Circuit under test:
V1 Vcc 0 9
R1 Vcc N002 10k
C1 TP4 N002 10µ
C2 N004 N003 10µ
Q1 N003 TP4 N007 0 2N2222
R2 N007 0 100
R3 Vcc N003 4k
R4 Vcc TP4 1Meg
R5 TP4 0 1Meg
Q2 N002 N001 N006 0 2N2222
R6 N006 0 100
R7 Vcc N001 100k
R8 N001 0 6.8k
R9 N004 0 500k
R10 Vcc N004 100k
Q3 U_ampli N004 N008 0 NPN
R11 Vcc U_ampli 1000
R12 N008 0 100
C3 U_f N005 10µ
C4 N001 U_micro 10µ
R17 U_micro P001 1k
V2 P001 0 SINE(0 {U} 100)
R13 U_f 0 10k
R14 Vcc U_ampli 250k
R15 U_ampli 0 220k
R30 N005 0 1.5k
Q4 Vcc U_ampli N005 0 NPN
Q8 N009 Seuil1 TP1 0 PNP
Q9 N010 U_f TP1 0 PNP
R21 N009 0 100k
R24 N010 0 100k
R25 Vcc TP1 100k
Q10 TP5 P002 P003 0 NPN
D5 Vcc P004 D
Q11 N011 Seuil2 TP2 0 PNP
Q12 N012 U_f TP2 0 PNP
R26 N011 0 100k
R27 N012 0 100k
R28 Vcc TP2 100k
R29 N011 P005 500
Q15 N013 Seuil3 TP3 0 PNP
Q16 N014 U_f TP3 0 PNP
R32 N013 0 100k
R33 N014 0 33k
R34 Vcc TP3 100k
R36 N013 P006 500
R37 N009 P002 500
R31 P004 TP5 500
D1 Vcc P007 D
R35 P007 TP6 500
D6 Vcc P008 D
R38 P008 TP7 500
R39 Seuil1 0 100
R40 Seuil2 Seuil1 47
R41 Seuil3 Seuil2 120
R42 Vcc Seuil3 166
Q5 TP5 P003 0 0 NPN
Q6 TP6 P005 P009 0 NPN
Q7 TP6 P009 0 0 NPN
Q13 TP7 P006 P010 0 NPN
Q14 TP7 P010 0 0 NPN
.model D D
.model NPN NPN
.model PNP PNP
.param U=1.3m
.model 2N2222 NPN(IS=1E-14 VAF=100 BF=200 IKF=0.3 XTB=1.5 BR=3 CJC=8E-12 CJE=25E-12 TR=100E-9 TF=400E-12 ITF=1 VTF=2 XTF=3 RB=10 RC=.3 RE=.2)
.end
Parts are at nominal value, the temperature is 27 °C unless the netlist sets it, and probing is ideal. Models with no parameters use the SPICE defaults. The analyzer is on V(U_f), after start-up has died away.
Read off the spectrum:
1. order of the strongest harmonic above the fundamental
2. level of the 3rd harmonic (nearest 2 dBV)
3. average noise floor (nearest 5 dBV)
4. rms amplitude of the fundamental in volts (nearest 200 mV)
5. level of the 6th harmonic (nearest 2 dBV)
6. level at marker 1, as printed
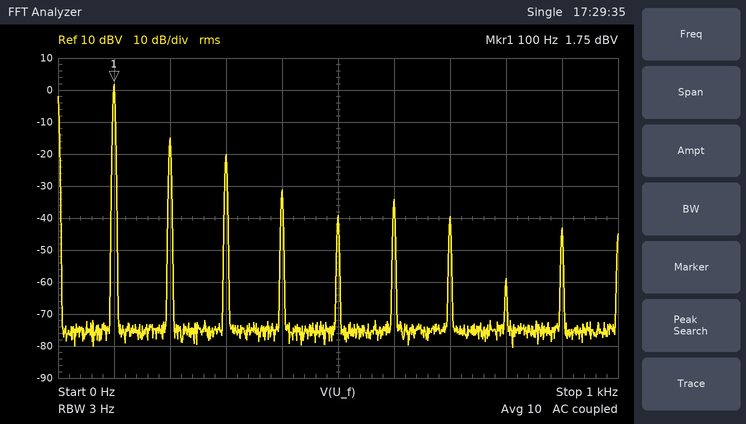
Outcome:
2
-20 dBV
-75 dBV
1.2 V
-34 dBV
1.75 dBV
